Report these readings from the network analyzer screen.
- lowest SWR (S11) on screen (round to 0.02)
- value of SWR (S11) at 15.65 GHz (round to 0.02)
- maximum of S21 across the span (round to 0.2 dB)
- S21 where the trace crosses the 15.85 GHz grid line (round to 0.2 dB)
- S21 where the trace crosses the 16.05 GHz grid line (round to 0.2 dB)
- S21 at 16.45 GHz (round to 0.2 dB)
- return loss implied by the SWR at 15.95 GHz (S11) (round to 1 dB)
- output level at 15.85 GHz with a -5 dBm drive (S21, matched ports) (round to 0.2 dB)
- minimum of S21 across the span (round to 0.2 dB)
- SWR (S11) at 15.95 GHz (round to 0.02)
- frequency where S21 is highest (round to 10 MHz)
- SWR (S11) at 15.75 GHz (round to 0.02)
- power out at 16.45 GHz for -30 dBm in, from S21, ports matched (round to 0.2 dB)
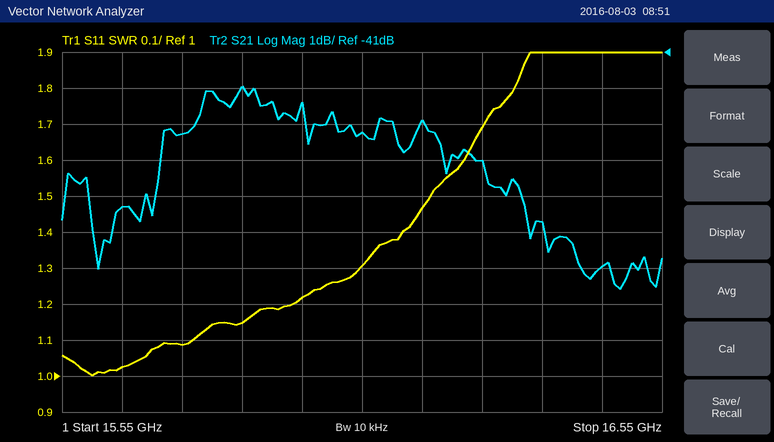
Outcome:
1.00
1.02
-42.0 dB
-42.0 dB
-43.2 dB
-47.0 dB
20 dB
-47.0 dBm
-47.6 dB
1.22
15.85 GHz
1.08
-77.0 dBm
